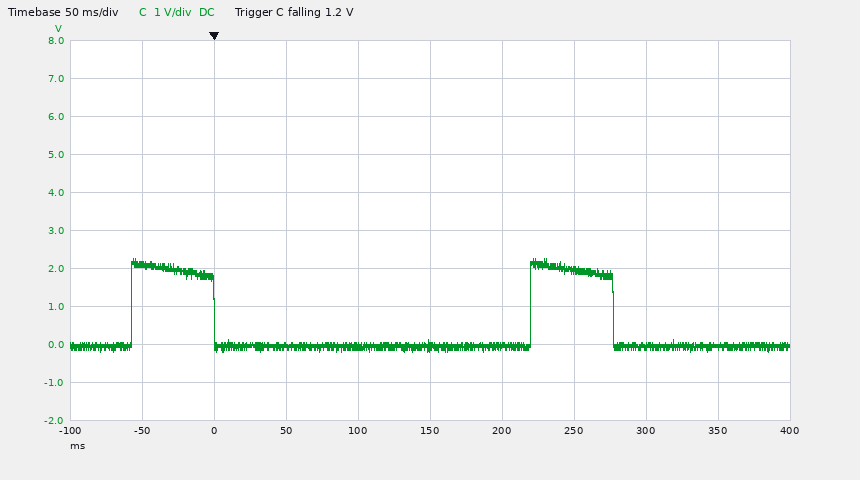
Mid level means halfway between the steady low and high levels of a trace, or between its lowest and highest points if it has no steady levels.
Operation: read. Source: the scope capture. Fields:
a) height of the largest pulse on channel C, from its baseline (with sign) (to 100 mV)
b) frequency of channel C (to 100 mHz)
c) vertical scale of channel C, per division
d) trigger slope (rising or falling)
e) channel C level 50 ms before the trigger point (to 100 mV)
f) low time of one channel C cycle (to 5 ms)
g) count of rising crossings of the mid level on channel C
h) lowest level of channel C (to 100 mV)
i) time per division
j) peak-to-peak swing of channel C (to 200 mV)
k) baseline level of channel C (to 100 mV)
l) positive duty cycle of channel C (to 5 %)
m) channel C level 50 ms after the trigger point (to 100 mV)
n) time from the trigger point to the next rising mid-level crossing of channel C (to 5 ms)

+2.3 V
3.6 Hz
1 V
falling
2.1 V
220 ms
2
-200 mV
50 ms
2.4 V
0.0 V
20 %
0.0 V
220 ms
